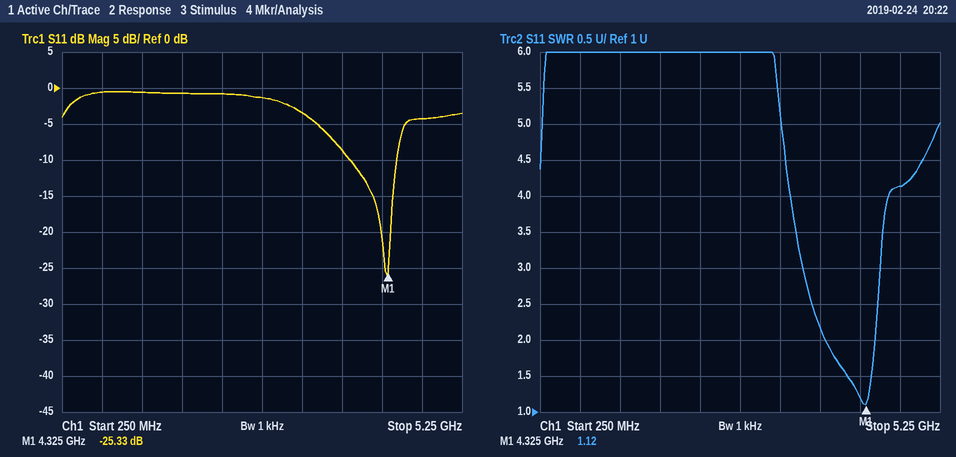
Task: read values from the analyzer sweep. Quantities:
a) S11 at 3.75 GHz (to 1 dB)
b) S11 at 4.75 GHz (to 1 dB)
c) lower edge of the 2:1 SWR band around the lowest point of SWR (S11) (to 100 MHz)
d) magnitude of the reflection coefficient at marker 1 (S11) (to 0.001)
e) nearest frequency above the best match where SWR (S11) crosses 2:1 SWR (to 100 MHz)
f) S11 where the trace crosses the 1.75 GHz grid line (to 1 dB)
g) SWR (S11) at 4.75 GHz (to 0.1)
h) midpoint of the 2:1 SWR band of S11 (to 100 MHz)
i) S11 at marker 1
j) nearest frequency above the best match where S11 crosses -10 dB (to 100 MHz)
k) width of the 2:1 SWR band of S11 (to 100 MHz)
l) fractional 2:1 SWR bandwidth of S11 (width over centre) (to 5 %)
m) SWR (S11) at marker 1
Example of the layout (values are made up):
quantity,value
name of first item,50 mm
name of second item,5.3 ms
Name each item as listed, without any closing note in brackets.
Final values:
quantity,value
S11 at 3.75 GHz,-9 dB
S11 at 4.75 GHz,-4 dB
lower edge of the 2:1 SWR band around the lowest point of SWR (S11),3.8 GHz
magnitude of the reflection coefficient at marker 1 (S11),0.054
nearest frequency above the best match where SWR (S11) crosses 2:1 SWR,4.4 GHz
S11 where the trace crosses the 1.75 GHz grid line,-1 dB
SWR (S11) at 4.75 GHz,4.1
midpoint of the 2:1 SWR band of S11,4.1 GHz
S11 at marker 1,-25.33 dB
nearest frequency above the best match where S11 crosses -10 dB,4.4 GHz
width of the 2:1 SWR band of S11,600 MHz
fractional 2:1 SWR bandwidth of S11 (width over centre),15 %
SWR (S11) at marker 1,1.12
